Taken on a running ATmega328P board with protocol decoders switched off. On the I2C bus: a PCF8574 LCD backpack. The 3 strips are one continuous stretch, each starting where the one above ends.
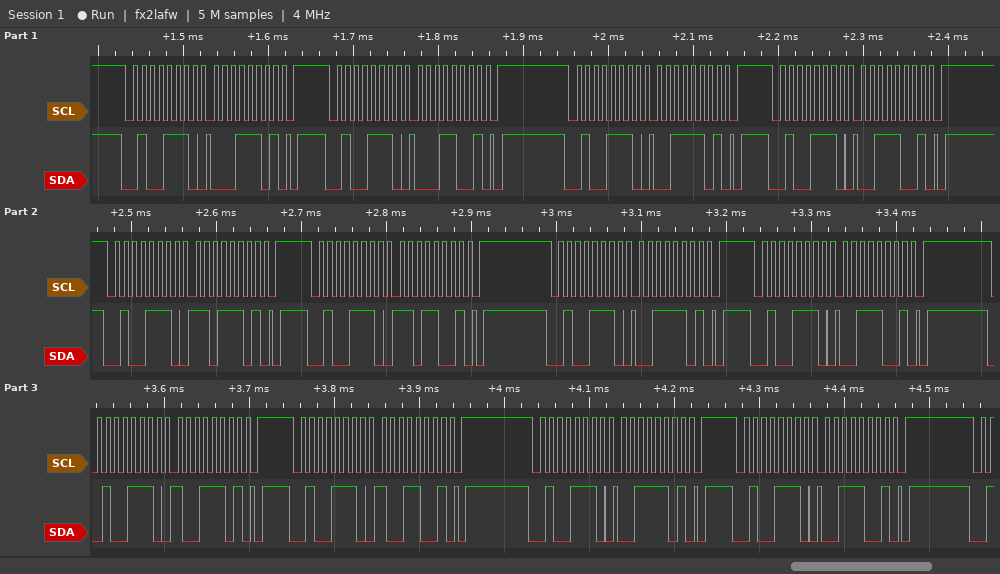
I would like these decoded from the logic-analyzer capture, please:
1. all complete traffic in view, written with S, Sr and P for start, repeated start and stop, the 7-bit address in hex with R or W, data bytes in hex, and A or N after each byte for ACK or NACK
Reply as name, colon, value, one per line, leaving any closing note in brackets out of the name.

all complete traffic in view, written with S, Sr and P for start, repeated start and stop, the 7-bit address in hex with R or W, data bytes in hex, and A or N after each byte for ACK or NACK: S 27W A 1D A P S 27W A 19 A P S 27W A 3D A P S 27W A 39 A P S 27W A DD A P S 27W A D9 A P S 27W A 3D A P S 27W A 39 A P S 27W A 9D A P S 27W A 99 A P S 27W A 3D A P S 27W A 39 A P
